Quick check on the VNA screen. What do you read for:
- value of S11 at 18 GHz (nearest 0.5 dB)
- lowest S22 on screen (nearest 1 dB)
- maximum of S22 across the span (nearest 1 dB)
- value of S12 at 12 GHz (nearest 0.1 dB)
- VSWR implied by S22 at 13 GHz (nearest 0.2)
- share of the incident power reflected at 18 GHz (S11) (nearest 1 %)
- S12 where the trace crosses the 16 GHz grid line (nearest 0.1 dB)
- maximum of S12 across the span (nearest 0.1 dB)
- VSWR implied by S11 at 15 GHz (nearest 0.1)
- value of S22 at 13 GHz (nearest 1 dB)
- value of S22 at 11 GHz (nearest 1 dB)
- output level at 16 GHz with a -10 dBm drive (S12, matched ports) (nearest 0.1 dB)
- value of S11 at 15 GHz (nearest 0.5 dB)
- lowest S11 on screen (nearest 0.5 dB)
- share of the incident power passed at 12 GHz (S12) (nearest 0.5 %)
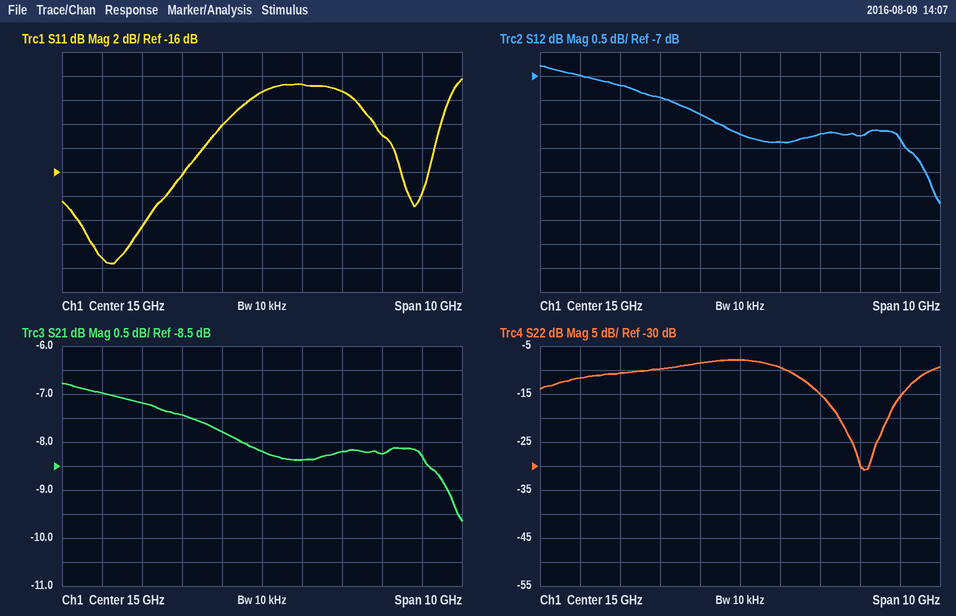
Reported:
-13.0 dB
-31 dB
-8 dB
-7.2 dB
2.0
5 %
-8.4 dB
-6.8 dB
2.0
-10 dB
-12 dB
-18.4 dBm
-9.5 dB
-23.5 dB
19.0 %
